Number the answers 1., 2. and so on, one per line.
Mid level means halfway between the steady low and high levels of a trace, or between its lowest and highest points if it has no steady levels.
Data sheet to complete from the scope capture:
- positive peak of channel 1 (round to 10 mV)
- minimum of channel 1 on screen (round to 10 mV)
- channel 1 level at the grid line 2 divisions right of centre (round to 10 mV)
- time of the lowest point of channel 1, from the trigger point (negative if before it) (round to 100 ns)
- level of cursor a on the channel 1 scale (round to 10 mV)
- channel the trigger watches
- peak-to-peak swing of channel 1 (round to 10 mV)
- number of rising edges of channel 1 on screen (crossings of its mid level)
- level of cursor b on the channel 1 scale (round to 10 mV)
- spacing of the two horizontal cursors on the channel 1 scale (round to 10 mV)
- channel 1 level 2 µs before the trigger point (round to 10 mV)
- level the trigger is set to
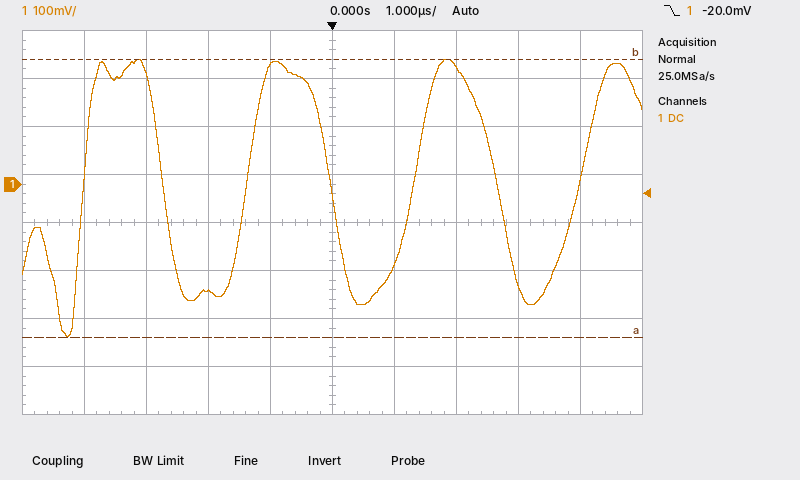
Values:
1. 260 mV
2. -320 mV
3. 240 mV
4. -4.3 µs
5. -320 mV
6. channel 1
7. 580 mV
8. 4
9. 260 mV
10. 580 mV
11. -220 mV
12. -20.0 mV
